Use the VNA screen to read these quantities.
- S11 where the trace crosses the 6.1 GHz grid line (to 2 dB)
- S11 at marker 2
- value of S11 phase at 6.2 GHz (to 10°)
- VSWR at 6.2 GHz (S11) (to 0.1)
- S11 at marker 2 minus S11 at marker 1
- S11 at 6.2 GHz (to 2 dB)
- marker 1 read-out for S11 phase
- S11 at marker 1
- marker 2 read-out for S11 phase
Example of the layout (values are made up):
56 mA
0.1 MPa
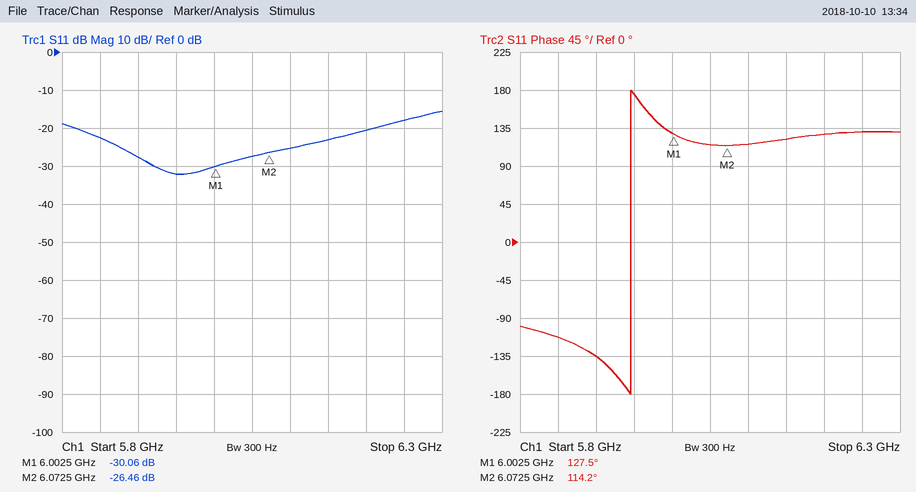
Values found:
-26 dB
-26.46 dB
130°
1.2
3.60 dB
-20 dB
127.5°
-30.06 dB
114.2°
